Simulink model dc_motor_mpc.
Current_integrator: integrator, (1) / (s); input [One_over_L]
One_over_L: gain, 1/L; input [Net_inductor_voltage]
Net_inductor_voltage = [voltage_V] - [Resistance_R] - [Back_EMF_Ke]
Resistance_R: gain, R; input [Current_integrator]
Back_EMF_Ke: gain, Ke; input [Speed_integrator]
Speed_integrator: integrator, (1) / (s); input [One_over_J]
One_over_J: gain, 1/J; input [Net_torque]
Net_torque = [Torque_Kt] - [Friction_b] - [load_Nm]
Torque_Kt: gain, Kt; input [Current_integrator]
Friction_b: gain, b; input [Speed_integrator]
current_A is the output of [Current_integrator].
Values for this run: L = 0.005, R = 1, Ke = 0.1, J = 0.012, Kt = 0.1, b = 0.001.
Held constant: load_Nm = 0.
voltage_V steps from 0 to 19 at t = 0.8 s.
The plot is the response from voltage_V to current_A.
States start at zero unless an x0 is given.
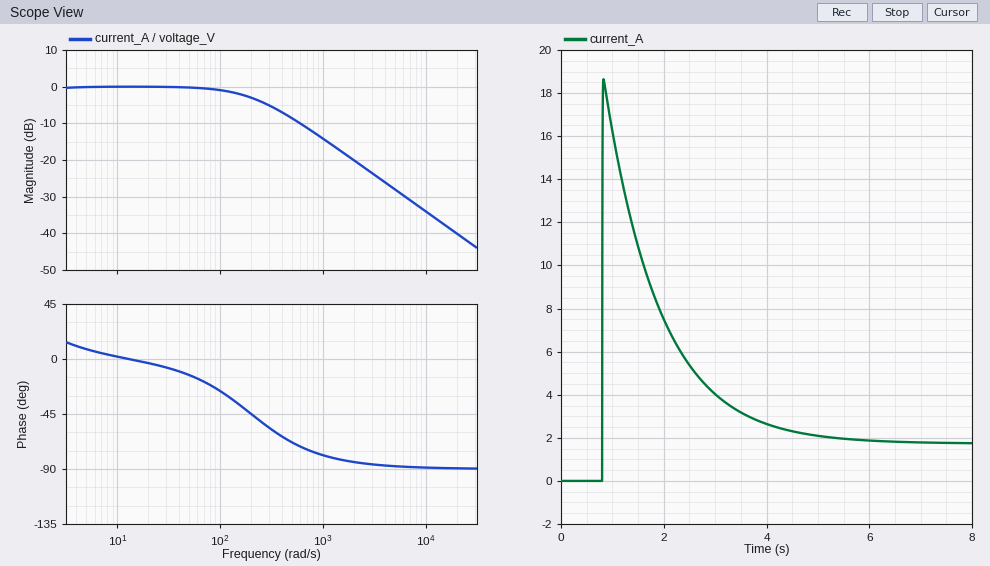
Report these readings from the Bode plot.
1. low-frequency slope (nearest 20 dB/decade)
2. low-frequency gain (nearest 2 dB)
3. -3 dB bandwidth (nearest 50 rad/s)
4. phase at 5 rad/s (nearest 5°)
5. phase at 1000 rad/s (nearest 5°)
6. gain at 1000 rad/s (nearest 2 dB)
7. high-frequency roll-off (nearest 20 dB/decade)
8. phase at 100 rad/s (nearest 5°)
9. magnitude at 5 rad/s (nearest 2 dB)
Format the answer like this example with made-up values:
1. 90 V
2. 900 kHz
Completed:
1. 0 dB/decade
2. 0 dB
3. 200 rad/s
4. 10°
5. -80°
6. -14 dB
7. -20 dB/decade
8. -25°
9. 0 dB
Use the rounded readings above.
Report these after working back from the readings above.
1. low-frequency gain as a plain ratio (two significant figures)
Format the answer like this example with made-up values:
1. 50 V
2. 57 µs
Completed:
1. 1.0
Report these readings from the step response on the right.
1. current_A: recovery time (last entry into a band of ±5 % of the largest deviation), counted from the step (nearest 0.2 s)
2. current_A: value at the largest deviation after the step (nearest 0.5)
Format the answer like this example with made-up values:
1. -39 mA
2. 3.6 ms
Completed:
1. 3.2 s
2. 18.5
